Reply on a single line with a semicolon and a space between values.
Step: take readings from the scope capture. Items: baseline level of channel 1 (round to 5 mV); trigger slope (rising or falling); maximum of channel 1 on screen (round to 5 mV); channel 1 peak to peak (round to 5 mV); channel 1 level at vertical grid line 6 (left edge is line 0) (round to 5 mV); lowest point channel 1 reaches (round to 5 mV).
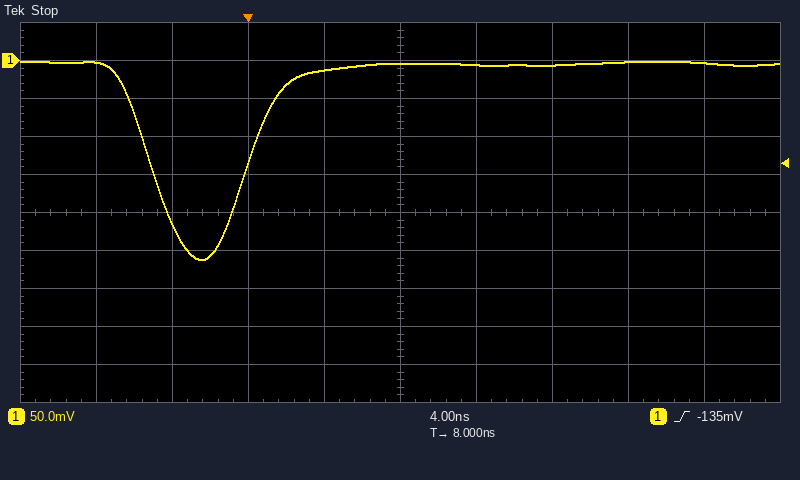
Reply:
-5 mV; rising; 0 mV; 260 mV; -5 mV; -260 mV
